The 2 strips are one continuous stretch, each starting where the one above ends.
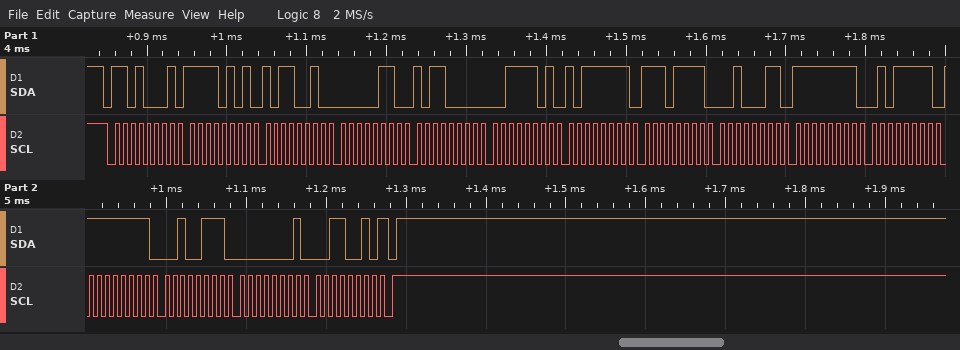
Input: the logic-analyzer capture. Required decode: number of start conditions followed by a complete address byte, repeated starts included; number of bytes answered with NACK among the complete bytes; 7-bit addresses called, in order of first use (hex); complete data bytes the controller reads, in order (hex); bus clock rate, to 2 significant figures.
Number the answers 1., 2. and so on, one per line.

1. 1
2. 1
3. 0x68
4. F5 B2 06 B0 3D BF EF 23 FF 5F FF 27 01 32
5. 100 kHz
